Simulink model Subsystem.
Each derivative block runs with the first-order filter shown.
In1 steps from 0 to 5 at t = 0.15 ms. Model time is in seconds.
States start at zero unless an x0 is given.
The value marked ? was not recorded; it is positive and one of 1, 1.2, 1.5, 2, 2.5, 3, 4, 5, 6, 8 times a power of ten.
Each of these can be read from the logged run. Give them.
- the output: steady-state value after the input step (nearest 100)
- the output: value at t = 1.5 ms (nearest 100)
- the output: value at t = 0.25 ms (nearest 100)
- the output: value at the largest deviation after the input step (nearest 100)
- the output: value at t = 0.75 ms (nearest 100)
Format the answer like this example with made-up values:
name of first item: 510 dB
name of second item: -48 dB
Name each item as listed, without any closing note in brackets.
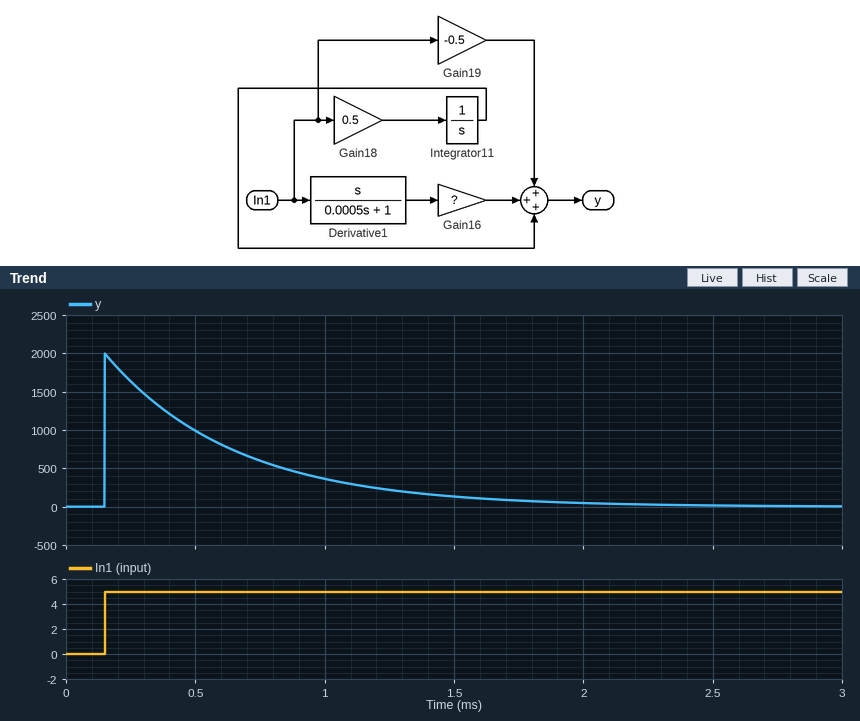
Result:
the output: steady-state value after the input step: 0
the output: value at t = 1.5 ms: 100
the output: value at t = 0.25 ms: 1600
the output: value at the largest deviation after the input step: 2000
the output: value at t = 0.75 ms: 600
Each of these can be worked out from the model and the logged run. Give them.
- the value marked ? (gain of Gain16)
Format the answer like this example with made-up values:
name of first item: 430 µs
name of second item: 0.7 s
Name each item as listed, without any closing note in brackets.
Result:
the value marked ?: 0.2
